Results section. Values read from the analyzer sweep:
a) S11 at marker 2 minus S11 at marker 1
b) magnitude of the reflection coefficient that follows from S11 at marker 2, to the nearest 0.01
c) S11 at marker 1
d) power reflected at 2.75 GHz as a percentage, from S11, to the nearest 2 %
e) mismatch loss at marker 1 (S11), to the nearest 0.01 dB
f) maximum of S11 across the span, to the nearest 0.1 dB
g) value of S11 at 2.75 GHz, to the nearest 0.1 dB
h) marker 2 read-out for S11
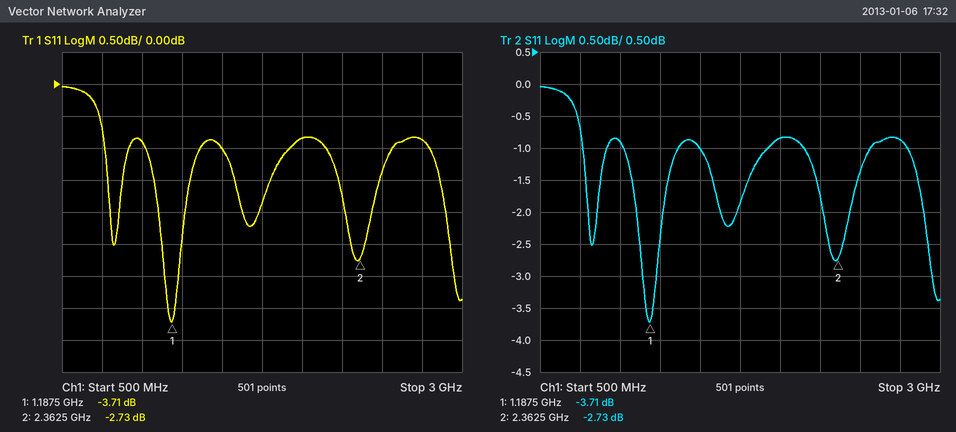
0.98 dB
0.73
-3.71 dB
82 %
2.41 dB
0.0 dB
-0.9 dB
-2.73 dB
